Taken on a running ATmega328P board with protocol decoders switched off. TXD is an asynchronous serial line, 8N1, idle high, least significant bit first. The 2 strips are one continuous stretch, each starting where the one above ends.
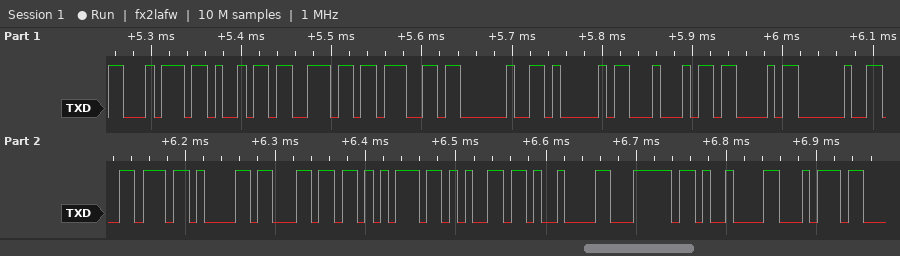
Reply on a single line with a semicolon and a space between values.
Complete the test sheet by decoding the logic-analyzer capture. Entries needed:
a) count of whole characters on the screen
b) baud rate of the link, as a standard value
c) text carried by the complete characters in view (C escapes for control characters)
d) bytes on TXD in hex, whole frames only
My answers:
18; 115200 baud; "ting ADC value\t|\tt"; 0x74 0x69 0x6E 0x67 0x20 0x41 0x44 0x43 0x20 0x76 0x61 0x6C 0x75 0x65 0x09 0x7C 0x09 0x74
